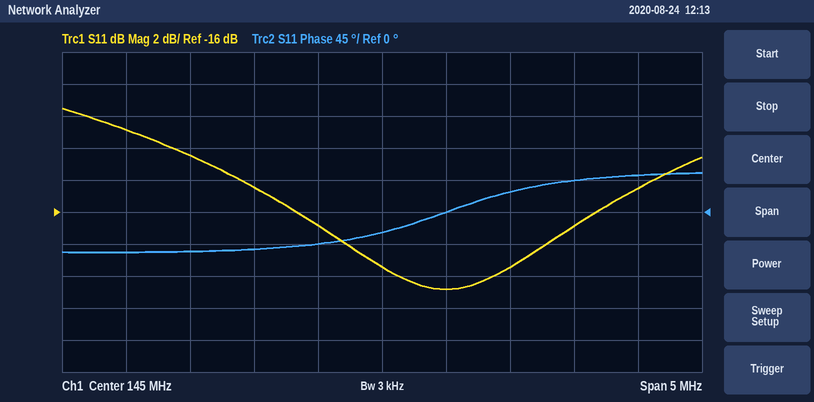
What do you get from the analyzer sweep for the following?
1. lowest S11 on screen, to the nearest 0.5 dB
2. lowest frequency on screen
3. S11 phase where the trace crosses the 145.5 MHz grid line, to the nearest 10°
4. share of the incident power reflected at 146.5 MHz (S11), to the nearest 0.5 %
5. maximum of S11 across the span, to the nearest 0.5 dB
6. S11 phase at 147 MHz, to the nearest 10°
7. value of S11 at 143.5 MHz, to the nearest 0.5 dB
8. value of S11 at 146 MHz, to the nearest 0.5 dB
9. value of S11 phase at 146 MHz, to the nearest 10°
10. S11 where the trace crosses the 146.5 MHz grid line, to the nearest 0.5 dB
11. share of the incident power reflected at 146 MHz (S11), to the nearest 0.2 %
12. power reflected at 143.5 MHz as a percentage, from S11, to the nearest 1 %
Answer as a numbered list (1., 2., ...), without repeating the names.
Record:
1. -21.0 dB
2. 142.5 MHz
3. 0°
4. 2.0 %
5. -9.5 dB
6. 50°
7. -12.5 dB
8. -19.5 dB
9. 30°
10. -17.0 dB
11. 1.2 %
12. 6 %
